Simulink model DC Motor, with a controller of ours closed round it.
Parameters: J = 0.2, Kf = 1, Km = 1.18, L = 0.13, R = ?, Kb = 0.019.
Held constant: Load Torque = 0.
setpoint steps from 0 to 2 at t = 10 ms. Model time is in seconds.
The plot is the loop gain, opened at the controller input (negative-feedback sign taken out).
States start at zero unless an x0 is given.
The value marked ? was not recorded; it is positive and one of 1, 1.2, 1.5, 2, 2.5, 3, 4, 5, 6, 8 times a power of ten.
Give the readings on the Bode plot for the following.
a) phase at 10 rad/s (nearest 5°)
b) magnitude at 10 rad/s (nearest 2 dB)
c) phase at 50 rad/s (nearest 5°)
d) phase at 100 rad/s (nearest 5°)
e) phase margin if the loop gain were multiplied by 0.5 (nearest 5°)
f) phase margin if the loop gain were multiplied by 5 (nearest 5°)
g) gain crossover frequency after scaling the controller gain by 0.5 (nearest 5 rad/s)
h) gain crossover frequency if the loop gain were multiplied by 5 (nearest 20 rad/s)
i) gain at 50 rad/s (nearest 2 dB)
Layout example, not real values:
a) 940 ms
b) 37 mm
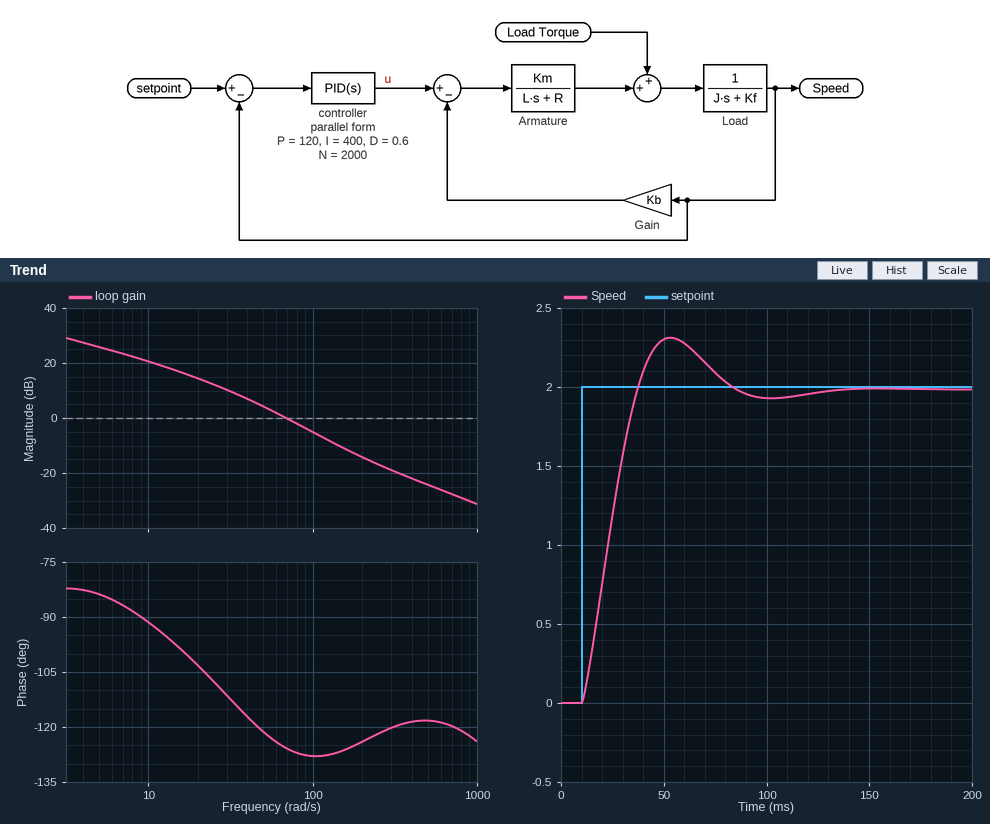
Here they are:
a) -90°
b) 20 dB
c) -120°
d) -130°
e) 60°
f) 55°
g) 45 rad/s
h) 200 rad/s
i) 4 dB
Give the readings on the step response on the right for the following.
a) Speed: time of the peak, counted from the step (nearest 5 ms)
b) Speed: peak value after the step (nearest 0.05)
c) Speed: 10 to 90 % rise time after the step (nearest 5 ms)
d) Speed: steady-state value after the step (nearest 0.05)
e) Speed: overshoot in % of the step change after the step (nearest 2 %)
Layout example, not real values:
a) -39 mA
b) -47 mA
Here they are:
a) 45 ms
b) 2.30
c) 20 ms
d) 2.00
e) 16 %
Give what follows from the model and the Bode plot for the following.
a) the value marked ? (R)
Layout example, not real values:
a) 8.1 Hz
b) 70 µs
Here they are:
a) 6
